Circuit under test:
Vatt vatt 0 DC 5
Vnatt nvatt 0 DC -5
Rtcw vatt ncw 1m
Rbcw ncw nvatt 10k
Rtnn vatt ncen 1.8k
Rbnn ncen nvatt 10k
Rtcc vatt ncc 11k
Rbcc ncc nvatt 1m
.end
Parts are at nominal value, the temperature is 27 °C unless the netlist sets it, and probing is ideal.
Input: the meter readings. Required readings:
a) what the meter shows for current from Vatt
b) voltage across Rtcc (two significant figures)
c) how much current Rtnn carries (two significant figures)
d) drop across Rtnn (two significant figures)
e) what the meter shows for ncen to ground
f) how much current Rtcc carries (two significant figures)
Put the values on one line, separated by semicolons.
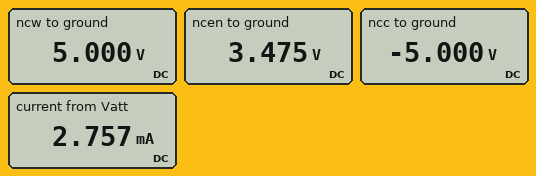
2.757 mA; 10 V; 850 µA; 1.5 V; 3.475 V; 910 µA
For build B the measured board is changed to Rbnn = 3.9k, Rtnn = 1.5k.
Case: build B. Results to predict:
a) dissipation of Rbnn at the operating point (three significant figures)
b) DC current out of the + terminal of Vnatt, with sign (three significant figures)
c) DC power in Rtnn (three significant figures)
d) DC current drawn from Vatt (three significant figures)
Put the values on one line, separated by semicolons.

13.4 mW; -3.76 mA; 5.14 mW; 3.76 mA
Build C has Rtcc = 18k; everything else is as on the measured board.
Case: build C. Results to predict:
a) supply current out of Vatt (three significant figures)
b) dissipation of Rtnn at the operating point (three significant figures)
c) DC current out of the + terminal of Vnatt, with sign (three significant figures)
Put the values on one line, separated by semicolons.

2.40 mA; 1.29 mW; -2.40 mA
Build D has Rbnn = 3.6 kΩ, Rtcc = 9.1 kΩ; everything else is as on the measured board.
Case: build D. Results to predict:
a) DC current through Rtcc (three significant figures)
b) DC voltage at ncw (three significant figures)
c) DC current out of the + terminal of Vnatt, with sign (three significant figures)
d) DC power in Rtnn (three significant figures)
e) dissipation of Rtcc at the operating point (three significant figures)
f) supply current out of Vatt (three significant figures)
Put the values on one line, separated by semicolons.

1.10 mA; 5.00 V; -3.95 mA; 6.17 mW; 11.0 mW; 3.95 mA
